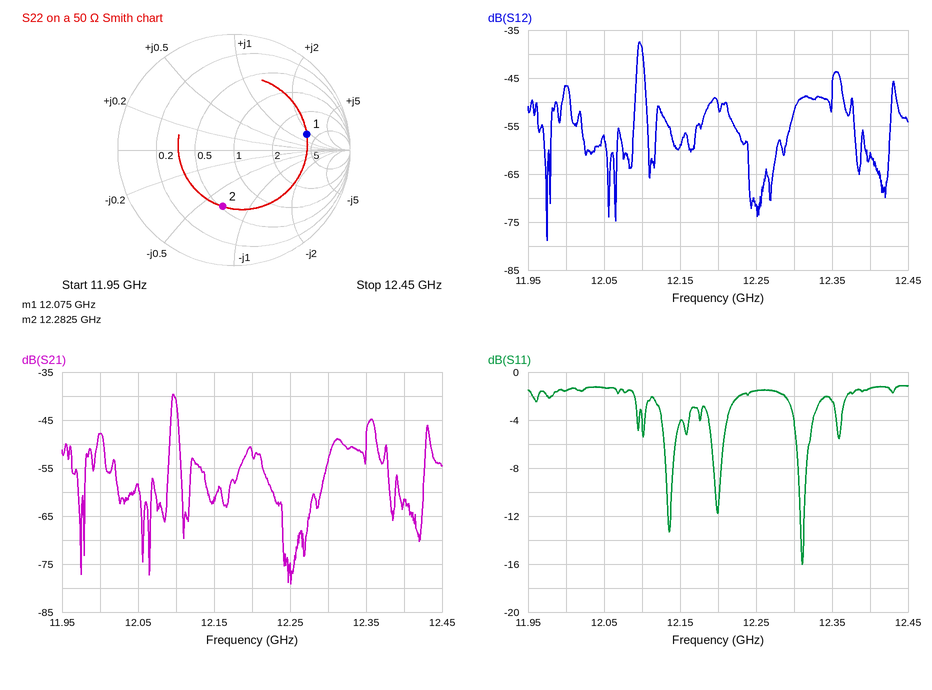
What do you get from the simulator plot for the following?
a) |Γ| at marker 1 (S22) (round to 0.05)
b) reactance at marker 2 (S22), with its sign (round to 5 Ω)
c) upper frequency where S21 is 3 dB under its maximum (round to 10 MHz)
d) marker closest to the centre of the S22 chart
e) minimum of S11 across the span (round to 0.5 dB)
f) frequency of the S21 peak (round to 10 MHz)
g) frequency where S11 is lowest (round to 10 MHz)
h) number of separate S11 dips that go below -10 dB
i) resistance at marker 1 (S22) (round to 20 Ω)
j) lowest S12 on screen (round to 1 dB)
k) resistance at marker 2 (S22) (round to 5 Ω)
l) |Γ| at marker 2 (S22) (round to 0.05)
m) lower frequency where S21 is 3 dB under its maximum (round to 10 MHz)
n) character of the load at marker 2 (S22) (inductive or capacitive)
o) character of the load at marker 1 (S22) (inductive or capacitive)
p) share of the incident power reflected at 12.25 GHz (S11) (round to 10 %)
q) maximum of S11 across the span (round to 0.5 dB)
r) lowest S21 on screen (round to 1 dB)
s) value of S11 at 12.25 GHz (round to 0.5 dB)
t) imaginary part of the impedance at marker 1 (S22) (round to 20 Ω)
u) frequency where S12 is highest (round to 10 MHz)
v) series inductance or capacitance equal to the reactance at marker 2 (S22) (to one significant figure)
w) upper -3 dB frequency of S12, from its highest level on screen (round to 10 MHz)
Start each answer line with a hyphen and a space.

- 0.65
- -35 Ω
- 12.10 GHz
- marker 2
- -16.0 dB
- 12.10 GHz
- 12.31 GHz
- 3
- 180 Ω
- -79 dB
- 25 Ω
- 0.50
- 12.09 GHz
- capacitive
- inductive
- 70 %
- -1.0 dB
- -79 dB
- -1.5 dB
- +80 Ω
- 12.10 GHz
- 400 fF
- 12.10 GHz
